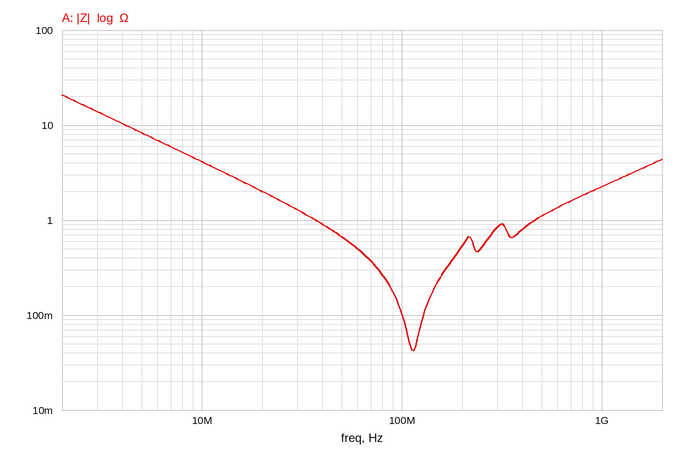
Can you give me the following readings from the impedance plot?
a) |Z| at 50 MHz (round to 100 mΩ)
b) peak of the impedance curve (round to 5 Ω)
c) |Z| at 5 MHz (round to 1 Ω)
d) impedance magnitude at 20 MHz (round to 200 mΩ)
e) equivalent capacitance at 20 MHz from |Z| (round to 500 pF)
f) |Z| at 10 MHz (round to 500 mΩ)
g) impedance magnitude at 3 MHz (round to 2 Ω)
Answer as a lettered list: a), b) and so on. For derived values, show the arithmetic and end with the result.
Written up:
a) 700 mΩ
b) 20 Ω
c) 8 Ω
d) 2.0 Ω
e) C = 1/(2π × 20 MHz × 2.0 Ω) ≈ 4.0 nF
f) 4.0 Ω
g) 14 Ω
